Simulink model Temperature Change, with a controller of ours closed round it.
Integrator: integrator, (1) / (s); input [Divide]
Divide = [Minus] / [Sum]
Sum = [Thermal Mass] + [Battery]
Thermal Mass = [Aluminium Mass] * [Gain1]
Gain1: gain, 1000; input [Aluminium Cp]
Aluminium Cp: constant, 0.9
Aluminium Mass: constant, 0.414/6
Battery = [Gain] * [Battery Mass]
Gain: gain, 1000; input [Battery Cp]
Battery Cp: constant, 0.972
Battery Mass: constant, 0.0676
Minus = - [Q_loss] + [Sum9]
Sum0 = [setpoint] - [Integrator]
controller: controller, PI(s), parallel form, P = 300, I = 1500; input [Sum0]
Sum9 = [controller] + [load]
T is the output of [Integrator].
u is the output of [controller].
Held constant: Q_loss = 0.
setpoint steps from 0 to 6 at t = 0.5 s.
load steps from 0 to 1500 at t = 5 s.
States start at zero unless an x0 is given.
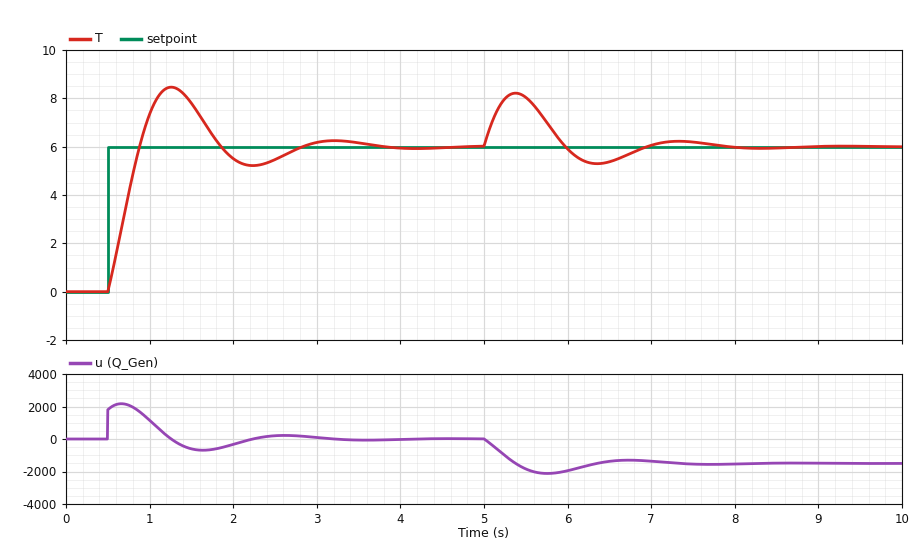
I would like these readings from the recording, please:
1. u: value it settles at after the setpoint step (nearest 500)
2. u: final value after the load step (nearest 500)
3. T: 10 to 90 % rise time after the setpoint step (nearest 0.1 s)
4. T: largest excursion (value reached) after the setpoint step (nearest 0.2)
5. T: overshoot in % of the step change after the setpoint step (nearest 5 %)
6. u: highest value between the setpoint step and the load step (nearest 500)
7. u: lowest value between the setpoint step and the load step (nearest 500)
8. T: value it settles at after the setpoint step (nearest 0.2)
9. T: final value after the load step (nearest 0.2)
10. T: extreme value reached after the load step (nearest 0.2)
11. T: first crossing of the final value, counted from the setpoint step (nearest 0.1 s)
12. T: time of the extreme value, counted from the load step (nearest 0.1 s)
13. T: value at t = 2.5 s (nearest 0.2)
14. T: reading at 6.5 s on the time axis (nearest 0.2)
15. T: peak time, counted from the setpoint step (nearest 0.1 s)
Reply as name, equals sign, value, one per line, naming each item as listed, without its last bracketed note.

u: value it settles at after the setpoint step = 0
u: final value after the load step = -1500
T: 10 to 90 % rise time after the setpoint step = 0.3 s
T: largest excursion (value reached) after the setpoint step = 8.4
T: overshoot in % of the step change after the setpoint step = 40 %
u: highest value between the setpoint step and the load step = 2000
u: lowest value between the setpoint step and the load step = -500
T: value it settles at after the setpoint step = 6.0
T: final value after the load step = 6.0
T: extreme value reached after the load step = 8.2
T: first crossing of the final value, counted from the setpoint step = 0.4 s
T: time of the extreme value, counted from the load step = 0.4 s
T: value at t = 2.5 s = 5.4
T: reading at 6.5 s on the time axis = 5.4
T: peak time, counted from the setpoint step = 0.8 s
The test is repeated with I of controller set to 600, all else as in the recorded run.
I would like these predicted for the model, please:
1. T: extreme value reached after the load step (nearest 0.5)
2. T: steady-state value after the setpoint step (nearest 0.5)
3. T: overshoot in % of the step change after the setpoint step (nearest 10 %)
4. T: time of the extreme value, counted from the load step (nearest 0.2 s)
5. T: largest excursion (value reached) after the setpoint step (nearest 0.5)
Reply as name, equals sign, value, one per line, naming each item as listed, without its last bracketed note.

T: extreme value reached after the load step = 9.0
T: steady-state value after the setpoint step = 6.0
T: overshoot in % of the step change after the setpoint step = 30 %
T: time of the extreme value, counted from the load step = 0.6 s
T: largest excursion (value reached) after the setpoint step = 7.5
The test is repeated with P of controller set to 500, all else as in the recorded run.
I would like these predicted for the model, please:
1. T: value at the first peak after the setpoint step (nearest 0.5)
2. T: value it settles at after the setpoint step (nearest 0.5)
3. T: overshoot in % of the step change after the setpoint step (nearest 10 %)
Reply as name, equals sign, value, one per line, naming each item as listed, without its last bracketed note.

T: value at the first peak after the setpoint step = 7.5
T: value it settles at after the setpoint step = 6.0
T: overshoot in % of the step change after the setpoint step = 30 %
